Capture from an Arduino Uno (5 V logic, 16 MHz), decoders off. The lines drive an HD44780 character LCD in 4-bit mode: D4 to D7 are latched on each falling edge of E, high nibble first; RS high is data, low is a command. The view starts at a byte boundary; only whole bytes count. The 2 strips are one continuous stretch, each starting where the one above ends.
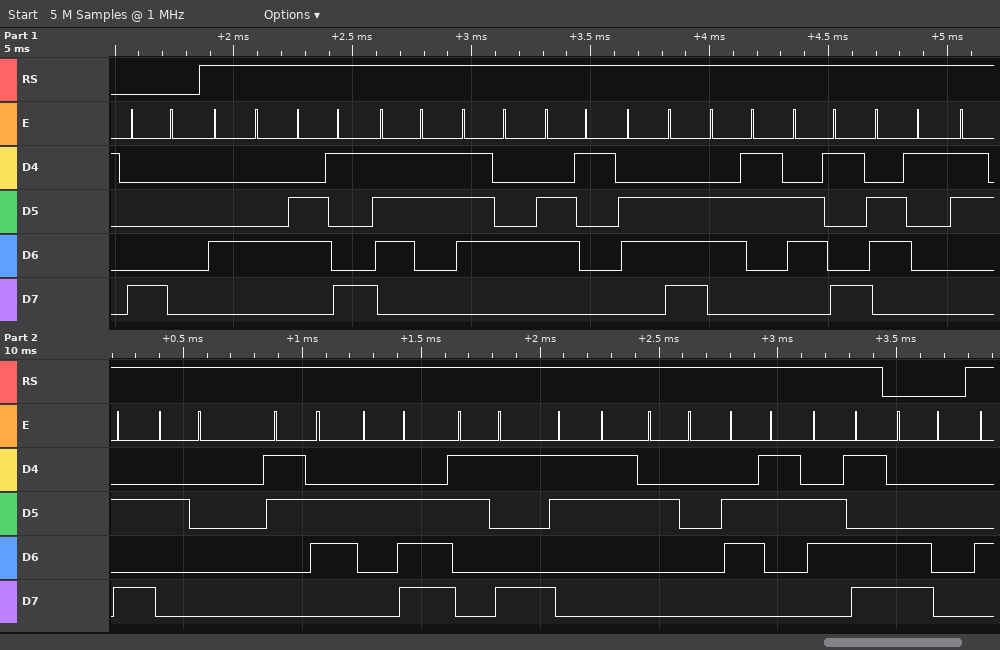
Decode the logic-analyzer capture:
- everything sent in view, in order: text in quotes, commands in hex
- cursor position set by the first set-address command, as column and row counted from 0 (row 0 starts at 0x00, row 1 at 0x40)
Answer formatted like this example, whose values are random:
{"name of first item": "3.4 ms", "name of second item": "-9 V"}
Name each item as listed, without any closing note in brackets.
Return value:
{"everything sent in view, in order: text in quotes, commands in hex": "0x80 \"Distancia: 6.93 cm\" 0xC0", "cursor position set by the first set-address command, as column and row counted from 0": "column 0, row 0"}
